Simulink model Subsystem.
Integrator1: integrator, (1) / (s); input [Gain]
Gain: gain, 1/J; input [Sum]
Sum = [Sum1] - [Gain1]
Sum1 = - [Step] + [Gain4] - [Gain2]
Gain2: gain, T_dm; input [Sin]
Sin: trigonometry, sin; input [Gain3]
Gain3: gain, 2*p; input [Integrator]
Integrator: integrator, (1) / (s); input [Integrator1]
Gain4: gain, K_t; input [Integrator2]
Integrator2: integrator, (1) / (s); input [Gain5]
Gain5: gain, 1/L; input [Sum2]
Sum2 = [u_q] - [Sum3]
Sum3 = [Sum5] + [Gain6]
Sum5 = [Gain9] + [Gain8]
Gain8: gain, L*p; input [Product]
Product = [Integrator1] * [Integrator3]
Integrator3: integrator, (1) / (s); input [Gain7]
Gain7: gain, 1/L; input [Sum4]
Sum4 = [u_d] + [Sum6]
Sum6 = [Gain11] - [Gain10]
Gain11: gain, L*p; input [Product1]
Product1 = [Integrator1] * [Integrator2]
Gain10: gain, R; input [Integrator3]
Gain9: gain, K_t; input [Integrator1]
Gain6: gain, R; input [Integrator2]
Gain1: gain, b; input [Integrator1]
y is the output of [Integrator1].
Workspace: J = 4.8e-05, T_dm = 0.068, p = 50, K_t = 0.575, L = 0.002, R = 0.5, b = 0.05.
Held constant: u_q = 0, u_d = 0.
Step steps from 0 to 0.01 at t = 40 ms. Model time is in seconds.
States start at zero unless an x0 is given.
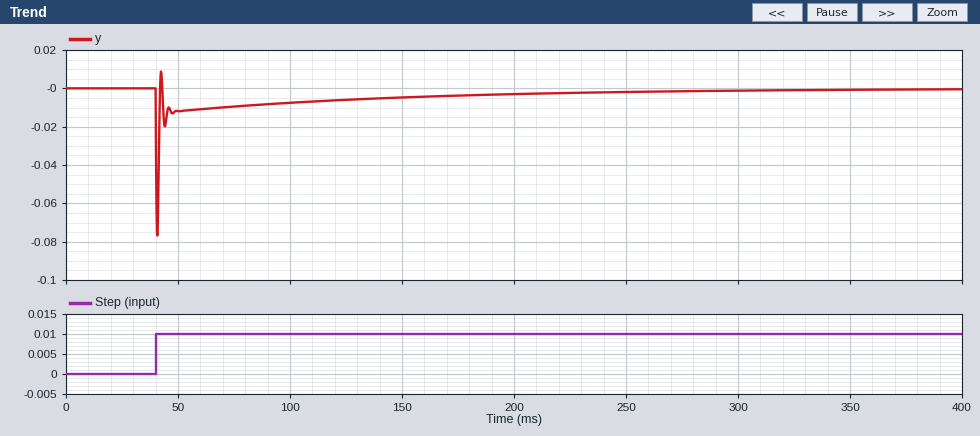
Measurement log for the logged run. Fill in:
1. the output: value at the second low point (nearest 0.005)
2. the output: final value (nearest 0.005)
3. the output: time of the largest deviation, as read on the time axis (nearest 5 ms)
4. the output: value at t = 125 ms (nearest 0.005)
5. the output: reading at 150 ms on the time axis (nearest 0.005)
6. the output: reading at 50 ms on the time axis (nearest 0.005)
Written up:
-0.020
0.000
40 ms
-0.005
-0.005
-0.010
